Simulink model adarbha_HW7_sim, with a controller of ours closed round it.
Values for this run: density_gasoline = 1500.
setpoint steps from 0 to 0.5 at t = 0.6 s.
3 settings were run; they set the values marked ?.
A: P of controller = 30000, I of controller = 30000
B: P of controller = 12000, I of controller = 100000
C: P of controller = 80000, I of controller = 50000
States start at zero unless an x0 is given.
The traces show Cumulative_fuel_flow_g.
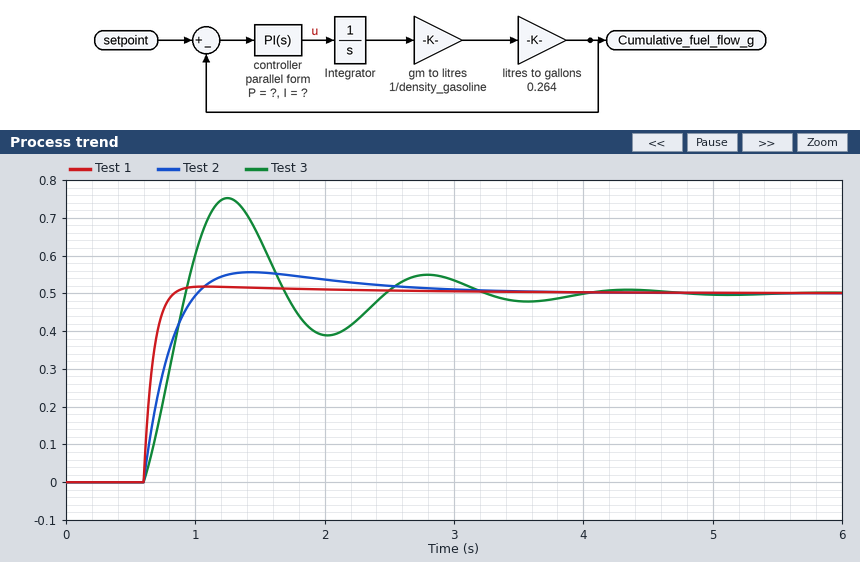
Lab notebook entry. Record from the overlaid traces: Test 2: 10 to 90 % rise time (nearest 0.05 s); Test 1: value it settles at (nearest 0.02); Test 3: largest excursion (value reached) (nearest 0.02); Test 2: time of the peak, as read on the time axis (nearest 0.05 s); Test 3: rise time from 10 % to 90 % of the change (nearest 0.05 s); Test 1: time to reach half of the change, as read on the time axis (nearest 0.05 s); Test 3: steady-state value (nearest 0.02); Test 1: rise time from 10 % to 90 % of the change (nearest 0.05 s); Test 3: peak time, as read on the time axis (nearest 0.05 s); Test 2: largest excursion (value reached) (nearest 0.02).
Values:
0.30 s
0.50
0.76
1.45 s
0.25 s
0.65 s
0.50
0.15 s
1.25 s
0.56
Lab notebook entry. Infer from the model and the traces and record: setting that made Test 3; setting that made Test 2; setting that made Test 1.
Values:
B
A
C
